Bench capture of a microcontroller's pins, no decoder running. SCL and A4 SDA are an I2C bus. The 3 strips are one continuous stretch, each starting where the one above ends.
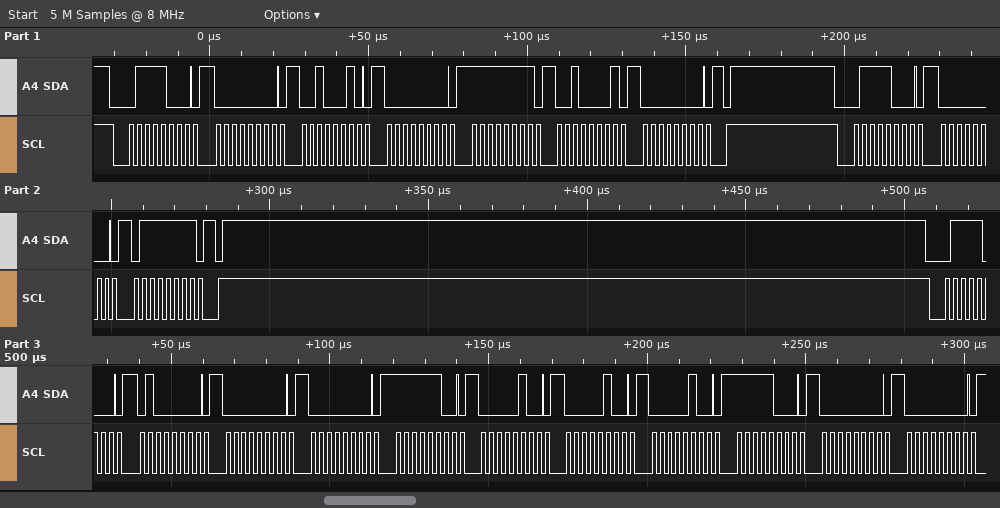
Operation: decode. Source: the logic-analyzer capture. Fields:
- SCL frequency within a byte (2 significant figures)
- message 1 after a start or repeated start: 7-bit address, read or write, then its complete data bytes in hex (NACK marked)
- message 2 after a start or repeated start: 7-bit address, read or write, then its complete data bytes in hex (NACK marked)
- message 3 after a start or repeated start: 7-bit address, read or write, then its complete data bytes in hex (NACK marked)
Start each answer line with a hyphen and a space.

- 400 kHz
- 0x3C write: 00 22 00 FF 21 00
- 0x3C write: 00 7F
- 0x3C write: 40 00 00 FC 04 04 04 F8 00 00
